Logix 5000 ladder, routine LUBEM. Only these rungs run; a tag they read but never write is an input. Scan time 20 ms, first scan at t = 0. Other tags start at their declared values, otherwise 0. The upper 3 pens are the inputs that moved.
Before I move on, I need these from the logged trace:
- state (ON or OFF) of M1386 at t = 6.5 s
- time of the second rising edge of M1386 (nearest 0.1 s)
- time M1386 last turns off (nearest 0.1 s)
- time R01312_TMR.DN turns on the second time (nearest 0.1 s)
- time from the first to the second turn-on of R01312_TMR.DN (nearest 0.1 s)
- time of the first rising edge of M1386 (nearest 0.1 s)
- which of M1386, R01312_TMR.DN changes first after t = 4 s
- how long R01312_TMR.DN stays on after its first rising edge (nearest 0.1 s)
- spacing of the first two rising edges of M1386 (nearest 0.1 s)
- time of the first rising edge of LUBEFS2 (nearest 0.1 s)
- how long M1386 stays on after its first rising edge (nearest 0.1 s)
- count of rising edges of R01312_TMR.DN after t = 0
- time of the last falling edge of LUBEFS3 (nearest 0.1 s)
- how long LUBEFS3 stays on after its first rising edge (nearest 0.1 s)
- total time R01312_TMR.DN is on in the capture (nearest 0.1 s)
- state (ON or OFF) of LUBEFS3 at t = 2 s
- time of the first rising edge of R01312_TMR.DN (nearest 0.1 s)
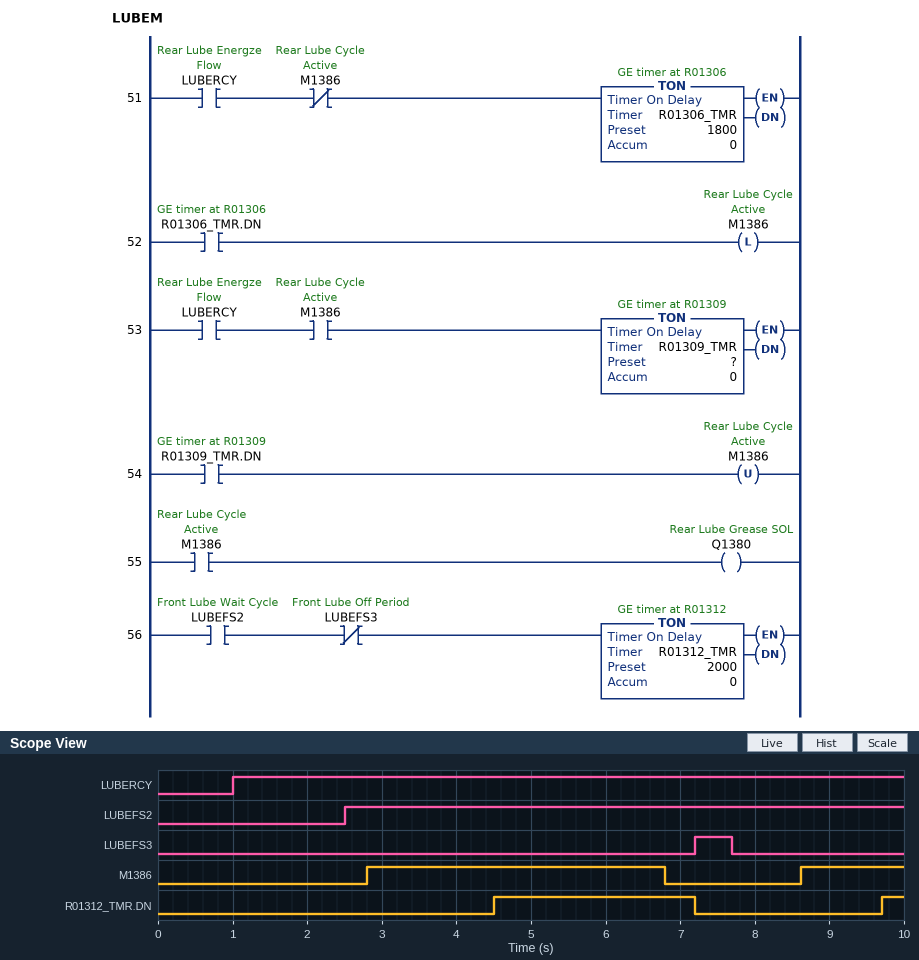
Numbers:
ON
8.6 s
6.8 s
9.7 s
5.2 s
2.8 s
R01312_TMR.DN
2.7 s
5.8 s
2.5 s
4.0 s
2
7.7 s
0.5 s
3.0 s
OFF
4.5 s
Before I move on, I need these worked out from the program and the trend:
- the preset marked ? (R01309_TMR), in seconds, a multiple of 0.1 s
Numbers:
4.0 s
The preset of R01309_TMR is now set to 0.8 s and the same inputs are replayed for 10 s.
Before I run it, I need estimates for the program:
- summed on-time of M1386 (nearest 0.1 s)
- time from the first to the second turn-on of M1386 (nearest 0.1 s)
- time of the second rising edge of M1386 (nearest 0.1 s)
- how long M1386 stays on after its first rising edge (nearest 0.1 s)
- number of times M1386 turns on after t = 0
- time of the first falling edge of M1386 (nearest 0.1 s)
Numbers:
2.4 s
2.6 s
5.4 s
0.8 s
3
3.6 s
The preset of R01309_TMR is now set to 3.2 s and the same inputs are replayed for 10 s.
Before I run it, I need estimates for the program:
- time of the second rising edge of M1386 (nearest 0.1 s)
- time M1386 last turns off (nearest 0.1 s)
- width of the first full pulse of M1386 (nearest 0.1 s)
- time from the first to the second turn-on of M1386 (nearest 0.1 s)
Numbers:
7.8 s
6.0 s
3.2 s
5.0 s
